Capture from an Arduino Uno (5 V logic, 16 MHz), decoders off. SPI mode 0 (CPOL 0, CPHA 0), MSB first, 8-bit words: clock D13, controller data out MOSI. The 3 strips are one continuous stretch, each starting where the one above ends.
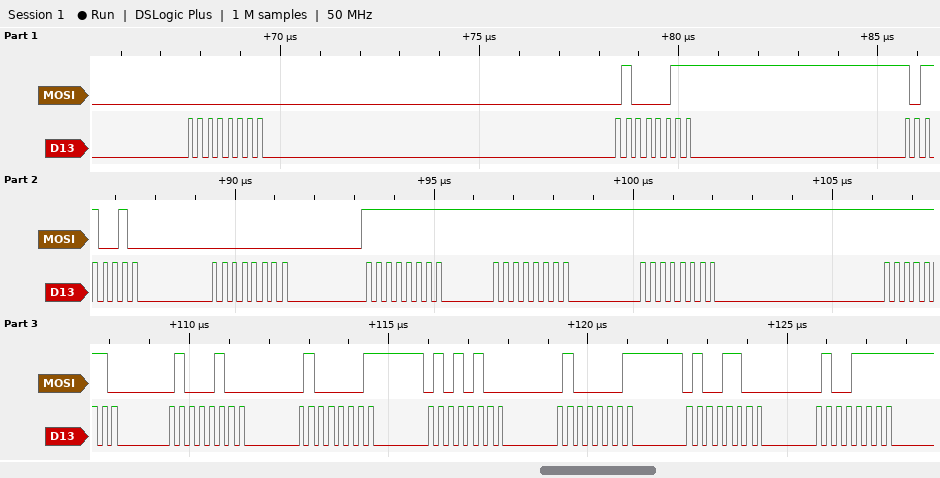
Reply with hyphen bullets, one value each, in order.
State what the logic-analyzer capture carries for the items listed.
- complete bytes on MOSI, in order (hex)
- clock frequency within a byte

- 00 43 B2 00 FF FF FF FE 44 41 54 41 4C 4F
- 4 MHz
